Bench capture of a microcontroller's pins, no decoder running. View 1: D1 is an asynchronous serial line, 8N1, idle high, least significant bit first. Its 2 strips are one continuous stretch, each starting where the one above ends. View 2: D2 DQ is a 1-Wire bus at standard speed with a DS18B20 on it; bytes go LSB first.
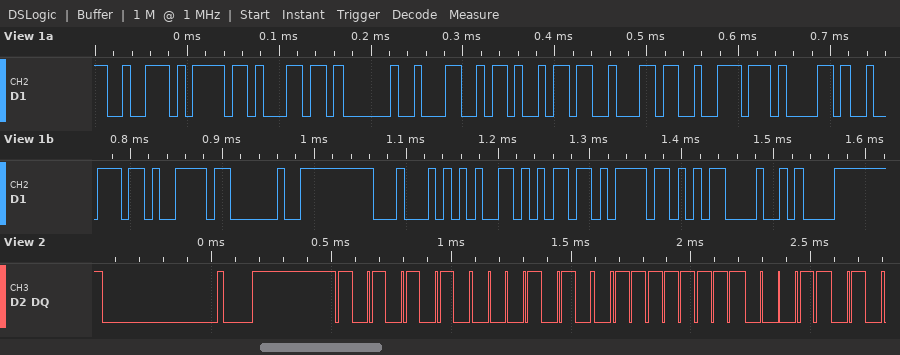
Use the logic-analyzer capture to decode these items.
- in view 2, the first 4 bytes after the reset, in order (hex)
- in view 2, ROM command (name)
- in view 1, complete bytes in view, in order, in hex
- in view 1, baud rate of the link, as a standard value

55 28 FF 58
Match ROM
72 6F 6C 20 4C 69 62 72 61 72 79 20 44 65 6D 6F 0D 0A
115200 baud
